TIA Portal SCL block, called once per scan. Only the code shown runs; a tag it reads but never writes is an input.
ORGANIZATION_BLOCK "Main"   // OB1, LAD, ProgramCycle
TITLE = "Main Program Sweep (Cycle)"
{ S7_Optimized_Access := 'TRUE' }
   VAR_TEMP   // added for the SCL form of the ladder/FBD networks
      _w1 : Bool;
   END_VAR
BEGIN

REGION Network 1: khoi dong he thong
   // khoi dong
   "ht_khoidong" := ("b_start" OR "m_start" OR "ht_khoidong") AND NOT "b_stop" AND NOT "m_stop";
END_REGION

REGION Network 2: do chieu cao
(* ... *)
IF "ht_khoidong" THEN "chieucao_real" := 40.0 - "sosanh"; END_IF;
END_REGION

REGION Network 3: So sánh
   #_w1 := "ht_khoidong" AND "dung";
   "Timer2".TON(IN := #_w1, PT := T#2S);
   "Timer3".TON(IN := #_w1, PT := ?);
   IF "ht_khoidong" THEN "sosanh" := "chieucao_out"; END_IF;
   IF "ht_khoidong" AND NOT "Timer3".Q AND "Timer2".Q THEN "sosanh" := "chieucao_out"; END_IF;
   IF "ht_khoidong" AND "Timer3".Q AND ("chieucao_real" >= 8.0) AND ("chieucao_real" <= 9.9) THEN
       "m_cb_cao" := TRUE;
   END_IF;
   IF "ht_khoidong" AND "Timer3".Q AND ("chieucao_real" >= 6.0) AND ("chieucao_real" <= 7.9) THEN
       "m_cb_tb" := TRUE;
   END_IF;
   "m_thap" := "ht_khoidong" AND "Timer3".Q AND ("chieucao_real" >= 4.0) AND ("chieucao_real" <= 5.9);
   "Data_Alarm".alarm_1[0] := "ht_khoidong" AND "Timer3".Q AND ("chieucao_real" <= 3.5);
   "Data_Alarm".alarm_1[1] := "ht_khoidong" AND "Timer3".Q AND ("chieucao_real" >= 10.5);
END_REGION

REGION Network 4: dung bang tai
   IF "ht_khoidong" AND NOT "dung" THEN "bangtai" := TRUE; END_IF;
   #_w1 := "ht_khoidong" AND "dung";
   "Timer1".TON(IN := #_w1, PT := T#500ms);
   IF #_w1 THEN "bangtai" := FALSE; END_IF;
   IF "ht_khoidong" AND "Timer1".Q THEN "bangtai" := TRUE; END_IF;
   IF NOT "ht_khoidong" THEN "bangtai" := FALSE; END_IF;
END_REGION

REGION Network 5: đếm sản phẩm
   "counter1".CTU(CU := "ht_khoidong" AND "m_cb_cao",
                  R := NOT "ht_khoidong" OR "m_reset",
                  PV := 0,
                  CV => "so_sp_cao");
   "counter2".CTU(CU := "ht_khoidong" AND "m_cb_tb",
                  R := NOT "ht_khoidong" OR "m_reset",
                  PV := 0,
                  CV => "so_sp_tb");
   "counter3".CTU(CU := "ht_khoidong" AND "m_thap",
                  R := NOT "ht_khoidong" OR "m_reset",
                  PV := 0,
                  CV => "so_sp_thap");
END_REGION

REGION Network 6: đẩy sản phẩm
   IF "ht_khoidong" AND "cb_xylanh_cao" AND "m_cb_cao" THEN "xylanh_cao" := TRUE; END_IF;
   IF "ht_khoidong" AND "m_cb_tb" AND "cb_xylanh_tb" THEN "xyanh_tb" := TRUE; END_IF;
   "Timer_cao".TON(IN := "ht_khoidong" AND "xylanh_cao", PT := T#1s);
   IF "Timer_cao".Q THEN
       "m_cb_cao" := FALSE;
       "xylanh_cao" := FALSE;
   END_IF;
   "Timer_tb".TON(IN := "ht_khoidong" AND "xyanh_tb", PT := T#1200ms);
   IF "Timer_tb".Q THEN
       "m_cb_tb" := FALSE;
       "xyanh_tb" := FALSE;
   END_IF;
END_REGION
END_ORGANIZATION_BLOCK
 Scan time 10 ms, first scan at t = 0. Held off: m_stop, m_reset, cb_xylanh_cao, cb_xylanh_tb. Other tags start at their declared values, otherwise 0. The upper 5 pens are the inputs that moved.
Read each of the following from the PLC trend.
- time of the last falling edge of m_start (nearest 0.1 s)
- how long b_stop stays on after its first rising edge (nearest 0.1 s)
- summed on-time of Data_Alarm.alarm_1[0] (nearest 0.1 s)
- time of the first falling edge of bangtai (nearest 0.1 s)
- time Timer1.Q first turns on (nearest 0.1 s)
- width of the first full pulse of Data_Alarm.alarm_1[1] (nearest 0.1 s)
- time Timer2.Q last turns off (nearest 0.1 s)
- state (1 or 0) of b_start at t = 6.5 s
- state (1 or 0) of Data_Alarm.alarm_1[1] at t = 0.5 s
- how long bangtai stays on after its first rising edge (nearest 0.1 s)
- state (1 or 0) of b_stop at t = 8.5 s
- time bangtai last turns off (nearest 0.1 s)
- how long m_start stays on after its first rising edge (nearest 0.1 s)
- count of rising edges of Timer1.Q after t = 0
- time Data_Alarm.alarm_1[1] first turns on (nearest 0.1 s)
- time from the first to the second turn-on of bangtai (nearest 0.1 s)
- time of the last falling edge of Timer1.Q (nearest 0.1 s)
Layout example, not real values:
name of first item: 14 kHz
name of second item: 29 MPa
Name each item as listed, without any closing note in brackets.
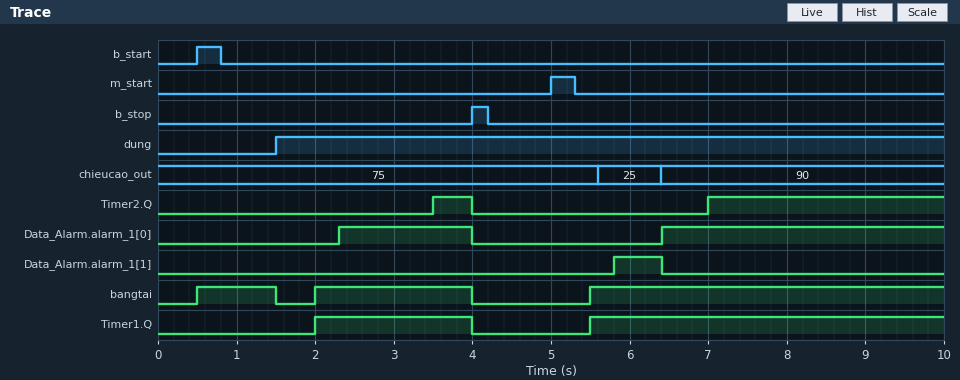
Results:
time of the last falling edge of m_start: 5.3 s
how long b_stop stays on after its first rising edge: 0.2 s
summed on-time of Data_Alarm.alarm_1[0]: 5.3 s
time of the first falling edge of bangtai: 1.5 s
time Timer1.Q first turns on: 2.0 s
width of the first full pulse of Data_Alarm.alarm_1[1]: 0.6 s
time Timer2.Q last turns off: 4.0 s
state (1 or 0) of b_start at t = 6.5 s: 0
state (1 or 0) of Data_Alarm.alarm_1[1] at t = 0.5 s: 0
how long bangtai stays on after its first rising edge: 1.0 s
state (1 or 0) of b_stop at t = 8.5 s: 0
time bangtai last turns off: 4.0 s
how long m_start stays on after its first rising edge: 0.3 s
count of rising edges of Timer1.Q after t = 0: 2
time Data_Alarm.alarm_1[1] first turns on: 5.8 s
time from the first to the second turn-on of bangtai: 1.5 s
time of the last falling edge of Timer1.Q: 4.0 s
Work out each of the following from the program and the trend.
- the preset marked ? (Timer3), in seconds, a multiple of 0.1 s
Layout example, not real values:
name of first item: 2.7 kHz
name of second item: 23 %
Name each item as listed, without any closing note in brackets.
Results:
the preset marked ? (Timer3), in seconds, a multiple of 0.1 s: 0.8 s
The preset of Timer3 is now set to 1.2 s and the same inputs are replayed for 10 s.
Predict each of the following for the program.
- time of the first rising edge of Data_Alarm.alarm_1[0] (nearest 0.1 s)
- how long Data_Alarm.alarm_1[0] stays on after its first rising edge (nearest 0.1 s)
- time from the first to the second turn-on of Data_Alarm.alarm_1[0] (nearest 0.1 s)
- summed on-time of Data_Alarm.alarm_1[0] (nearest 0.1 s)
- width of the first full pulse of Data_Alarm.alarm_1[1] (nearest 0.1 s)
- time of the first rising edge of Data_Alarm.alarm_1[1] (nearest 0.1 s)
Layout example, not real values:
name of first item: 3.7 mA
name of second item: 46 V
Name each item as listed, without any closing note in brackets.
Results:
time of the first rising edge of Data_Alarm.alarm_1[0]: 2.7 s
how long Data_Alarm.alarm_1[0] stays on after its first rising edge: 1.3 s
time from the first to the second turn-on of Data_Alarm.alarm_1[0]: 3.7 s
summed on-time of Data_Alarm.alarm_1[0]: 4.9 s
width of the first full pulse of Data_Alarm.alarm_1[1]: 0.2 s
time of the first rising edge of Data_Alarm.alarm_1[1]: 6.2 s
